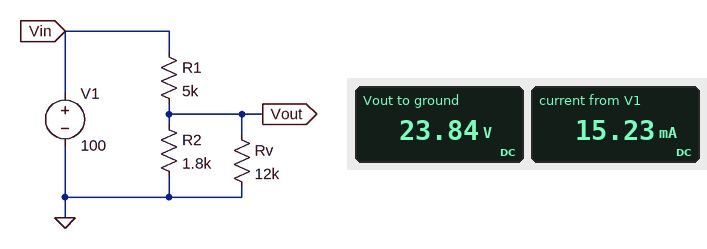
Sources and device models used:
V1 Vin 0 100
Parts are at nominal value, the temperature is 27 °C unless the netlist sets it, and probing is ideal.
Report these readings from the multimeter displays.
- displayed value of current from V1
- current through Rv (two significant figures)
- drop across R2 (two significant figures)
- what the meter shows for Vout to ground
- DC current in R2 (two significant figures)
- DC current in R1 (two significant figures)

15.23 mA
2.0 mA
24 V
23.84 V
13 mA
15 mA
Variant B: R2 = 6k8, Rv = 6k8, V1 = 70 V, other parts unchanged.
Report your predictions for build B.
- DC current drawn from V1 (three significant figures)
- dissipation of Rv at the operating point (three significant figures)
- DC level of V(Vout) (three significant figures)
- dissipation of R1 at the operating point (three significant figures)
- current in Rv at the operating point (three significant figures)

8.33 mA
118 mW
28.3 V
347 mW
4.17 mA
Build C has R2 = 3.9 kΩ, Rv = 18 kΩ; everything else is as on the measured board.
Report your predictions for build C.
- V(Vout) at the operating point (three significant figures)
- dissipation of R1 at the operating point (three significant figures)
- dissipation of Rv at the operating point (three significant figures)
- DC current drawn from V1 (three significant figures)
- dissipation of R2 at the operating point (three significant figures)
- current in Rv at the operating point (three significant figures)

39.1 V
743 mW
84.8 mW
12.2 mA
391 mW
2.17 mA
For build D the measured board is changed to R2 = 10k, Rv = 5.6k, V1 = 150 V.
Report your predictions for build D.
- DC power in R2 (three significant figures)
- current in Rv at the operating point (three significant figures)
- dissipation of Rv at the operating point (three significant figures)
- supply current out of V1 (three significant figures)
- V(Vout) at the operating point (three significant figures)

393 mW
11.2 mA
702 mW
17.5 mA
62.7 V
